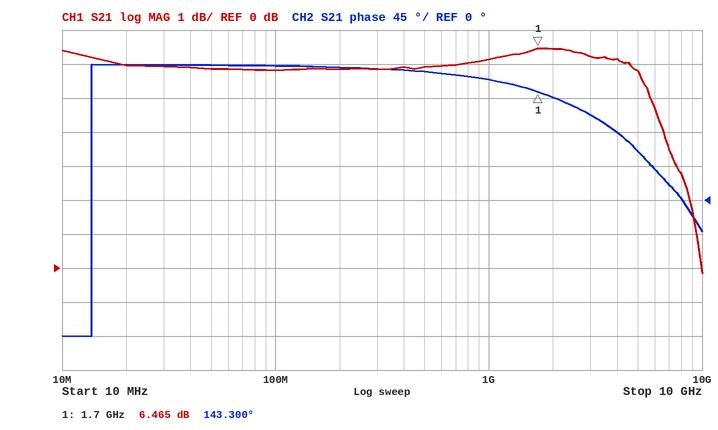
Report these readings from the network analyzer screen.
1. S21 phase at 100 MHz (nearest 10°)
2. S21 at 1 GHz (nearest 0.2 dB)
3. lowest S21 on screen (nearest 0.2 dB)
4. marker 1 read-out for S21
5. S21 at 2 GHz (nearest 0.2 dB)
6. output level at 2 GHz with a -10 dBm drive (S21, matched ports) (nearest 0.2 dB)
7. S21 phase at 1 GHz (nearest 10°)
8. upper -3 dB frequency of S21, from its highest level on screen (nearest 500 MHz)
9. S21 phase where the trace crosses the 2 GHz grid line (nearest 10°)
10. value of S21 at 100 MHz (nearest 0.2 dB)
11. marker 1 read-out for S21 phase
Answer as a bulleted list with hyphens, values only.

- 180°
- 6.2 dB
- -0.2 dB
- 6.465 dB
- 6.4 dB
- -3.6 dBm
- 160°
- 7.0 GHz
- 140°
- 5.8 dB
- 143.300°
